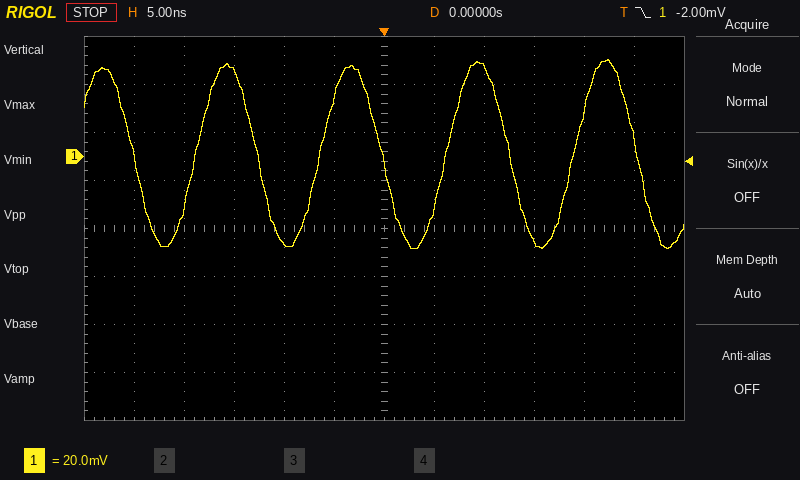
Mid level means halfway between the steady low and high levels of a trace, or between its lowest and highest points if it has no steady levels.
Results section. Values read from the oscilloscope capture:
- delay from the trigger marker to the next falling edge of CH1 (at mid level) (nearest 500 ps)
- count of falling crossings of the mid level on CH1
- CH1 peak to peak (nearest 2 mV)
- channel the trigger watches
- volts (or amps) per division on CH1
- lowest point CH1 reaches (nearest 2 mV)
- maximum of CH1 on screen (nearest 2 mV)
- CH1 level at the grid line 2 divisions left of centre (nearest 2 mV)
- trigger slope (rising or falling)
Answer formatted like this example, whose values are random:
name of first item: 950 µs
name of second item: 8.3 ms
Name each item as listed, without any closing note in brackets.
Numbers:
delay from the trigger marker to the next falling edge of CH1 (at mid level): 12.5 ns
count of falling crossings of the mid level on CH1: 5
CH1 peak to peak: 78 mV
channel the trigger watches: CH1
volts (or amps) per division on CH1: 20 mV
lowest point CH1 reaches: -38 mV
maximum of CH1 on screen: 40 mV
CH1 level at the grid line 2 divisions left of centre: -36 mV
trigger slope: falling
